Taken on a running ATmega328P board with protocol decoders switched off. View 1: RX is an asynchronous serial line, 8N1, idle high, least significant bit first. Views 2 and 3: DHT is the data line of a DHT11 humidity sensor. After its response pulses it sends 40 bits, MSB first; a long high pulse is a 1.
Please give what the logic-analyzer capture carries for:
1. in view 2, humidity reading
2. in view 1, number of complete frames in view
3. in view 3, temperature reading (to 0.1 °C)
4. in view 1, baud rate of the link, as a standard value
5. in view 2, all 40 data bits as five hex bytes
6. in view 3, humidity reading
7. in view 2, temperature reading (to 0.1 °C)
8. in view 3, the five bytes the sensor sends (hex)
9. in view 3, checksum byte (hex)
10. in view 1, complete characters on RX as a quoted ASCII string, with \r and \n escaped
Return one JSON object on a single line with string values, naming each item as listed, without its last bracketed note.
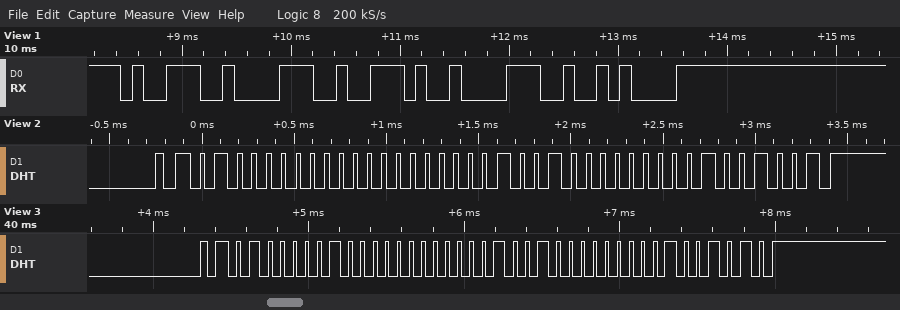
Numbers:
{"in view 2, humidity reading": "64 %", "in view 1, number of complete frames in view": "5", "in view 3, temperature reading": "9.0 °C", "in view 1, baud rate of the link, as a standard value": "9600 baud", "in view 2, all 40 data bits as five hex bytes": "40 00 09 00 49", "in view 3, humidity reading": "65 %", "in view 2, temperature reading": "9.0 °C", "in view 3, the five bytes the sensor sends": "41 00 09 00 4A", "in view 3, checksum byte": "0x4A", "in view 1, complete characters on RX as a quoted ASCII string, with \\r and \\n escaped": "\"98.8\\n\""}
